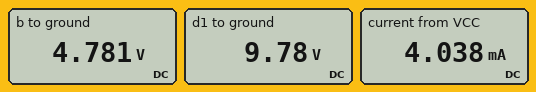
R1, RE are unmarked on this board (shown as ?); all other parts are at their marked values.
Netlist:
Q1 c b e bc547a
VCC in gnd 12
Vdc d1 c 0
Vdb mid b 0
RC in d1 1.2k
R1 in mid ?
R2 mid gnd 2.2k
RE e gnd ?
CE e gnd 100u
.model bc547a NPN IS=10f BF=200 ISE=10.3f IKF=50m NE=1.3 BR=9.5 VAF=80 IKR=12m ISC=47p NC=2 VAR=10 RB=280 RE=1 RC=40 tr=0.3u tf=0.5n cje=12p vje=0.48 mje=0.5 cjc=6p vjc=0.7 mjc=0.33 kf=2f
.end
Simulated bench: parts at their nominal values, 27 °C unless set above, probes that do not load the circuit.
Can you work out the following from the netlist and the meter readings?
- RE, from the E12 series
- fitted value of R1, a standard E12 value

2.2 kΩ
3.3 kΩ
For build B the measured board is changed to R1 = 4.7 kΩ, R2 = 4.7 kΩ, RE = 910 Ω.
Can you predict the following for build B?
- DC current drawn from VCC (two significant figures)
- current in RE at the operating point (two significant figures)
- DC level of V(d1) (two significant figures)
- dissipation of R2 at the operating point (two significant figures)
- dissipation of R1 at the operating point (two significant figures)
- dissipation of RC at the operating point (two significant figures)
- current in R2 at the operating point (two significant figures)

6.8 mA
5.6 mA
5.4 V
7.2 mW
8.1 mW
36 mW
1.2 mA
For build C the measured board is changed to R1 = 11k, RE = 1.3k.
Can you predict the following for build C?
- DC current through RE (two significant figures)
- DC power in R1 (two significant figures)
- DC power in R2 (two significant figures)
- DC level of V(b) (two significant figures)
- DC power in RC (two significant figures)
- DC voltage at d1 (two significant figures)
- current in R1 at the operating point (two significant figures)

1.0 mA
9.1 mW
1.8 mW
2.0 V
1.2 mW
11 V
910 µA
